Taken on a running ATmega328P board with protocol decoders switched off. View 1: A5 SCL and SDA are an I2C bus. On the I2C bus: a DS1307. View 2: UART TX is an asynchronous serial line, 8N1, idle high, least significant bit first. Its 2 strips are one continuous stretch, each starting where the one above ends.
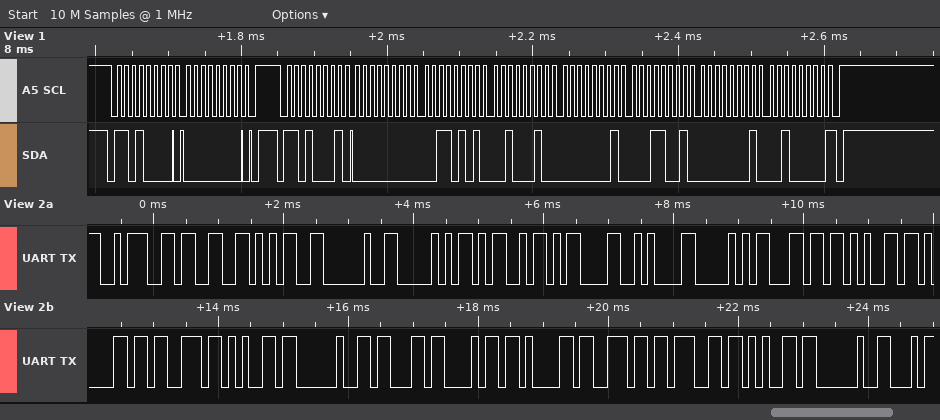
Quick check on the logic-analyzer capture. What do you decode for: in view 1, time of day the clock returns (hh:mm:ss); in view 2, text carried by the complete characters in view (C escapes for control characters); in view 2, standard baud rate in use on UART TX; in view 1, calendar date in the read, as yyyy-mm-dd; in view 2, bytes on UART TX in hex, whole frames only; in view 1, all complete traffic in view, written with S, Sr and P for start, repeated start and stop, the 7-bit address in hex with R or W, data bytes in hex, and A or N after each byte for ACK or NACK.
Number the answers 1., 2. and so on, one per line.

1. 22:35:00
2. ":35 PM\r\nPlease change "
3. 9600 baud
4. 2020-01-19
5. 3A 33 35 20 50 4D 0D 0A 50 6C 65 61 73 65 20 63 68 61 6E 67 65 20
6. S 68W A 00 A P S 68R A 00 A 35 A 22 A 01 A 19 A 01 A 20 N P
